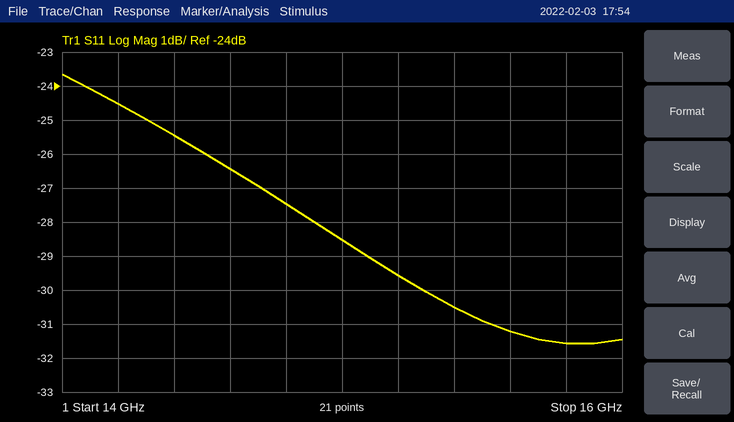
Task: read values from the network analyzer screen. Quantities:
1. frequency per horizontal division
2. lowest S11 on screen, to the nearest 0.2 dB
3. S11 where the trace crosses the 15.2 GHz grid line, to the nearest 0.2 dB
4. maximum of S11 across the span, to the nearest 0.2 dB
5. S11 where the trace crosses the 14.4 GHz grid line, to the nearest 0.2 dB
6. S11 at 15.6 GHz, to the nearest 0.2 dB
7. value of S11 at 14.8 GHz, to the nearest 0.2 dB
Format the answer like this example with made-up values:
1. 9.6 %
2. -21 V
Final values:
1. 200 MHz
2. -31.6 dB
3. -29.6 dB
4. -23.6 dB
5. -25.4 dB
6. -31.2 dB
7. -27.4 dB
